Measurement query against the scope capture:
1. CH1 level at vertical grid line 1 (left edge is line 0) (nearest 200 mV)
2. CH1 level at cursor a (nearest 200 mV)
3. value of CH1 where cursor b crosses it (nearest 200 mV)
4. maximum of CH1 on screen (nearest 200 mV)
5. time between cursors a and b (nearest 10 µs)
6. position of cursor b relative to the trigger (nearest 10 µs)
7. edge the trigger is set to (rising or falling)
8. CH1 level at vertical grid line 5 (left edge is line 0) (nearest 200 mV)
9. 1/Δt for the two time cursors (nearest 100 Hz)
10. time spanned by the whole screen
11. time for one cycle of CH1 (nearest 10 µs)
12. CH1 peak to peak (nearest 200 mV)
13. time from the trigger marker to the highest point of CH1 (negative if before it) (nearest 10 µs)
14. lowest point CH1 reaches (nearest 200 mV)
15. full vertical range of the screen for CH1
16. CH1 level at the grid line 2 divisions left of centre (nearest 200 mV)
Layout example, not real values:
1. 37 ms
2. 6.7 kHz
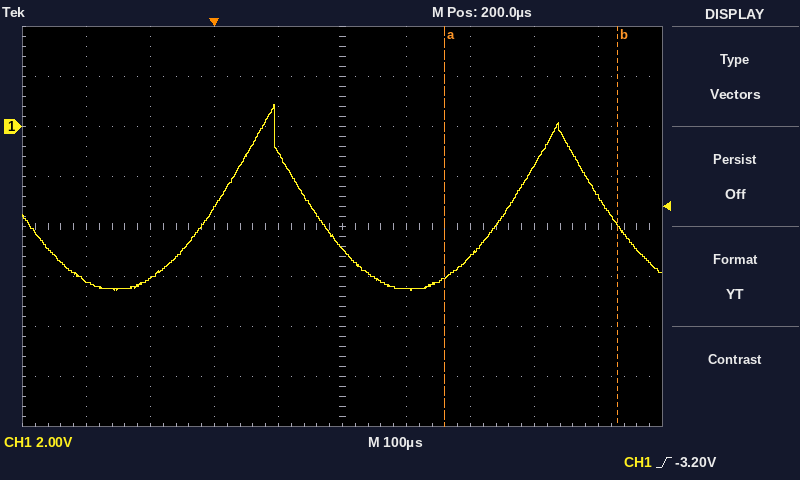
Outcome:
1. -6.2 V
2. -6.0 V
3. -4.0 V
4. 800 mV
5. 270 µs
6. +630 µs
7. rising
8. -4.8 V
9. 3.7 kHz
10. 1 ms
11. 460 µs
12. 7.4 V
13. +90 µs
14. -6.6 V
15. 16 V
16. -3.2 V
